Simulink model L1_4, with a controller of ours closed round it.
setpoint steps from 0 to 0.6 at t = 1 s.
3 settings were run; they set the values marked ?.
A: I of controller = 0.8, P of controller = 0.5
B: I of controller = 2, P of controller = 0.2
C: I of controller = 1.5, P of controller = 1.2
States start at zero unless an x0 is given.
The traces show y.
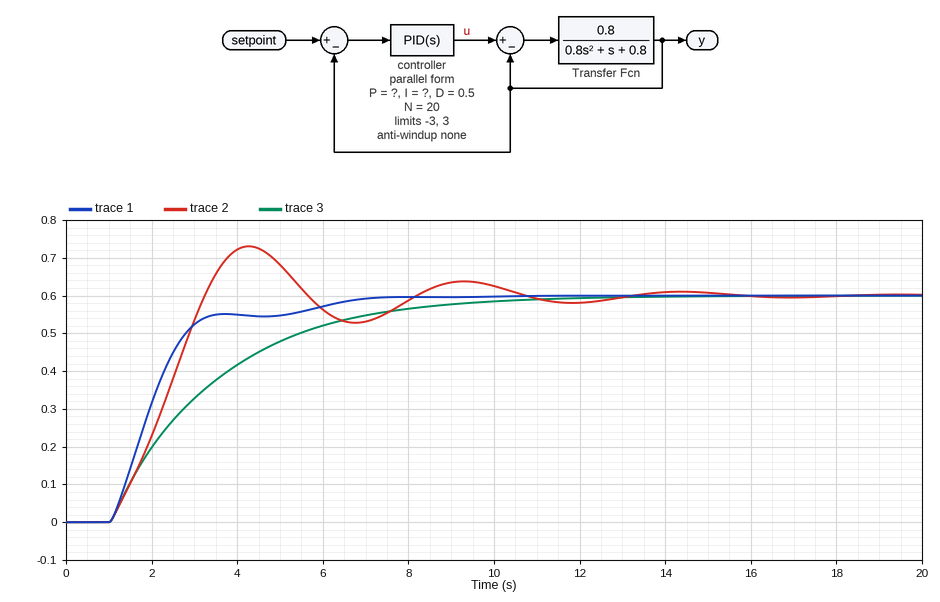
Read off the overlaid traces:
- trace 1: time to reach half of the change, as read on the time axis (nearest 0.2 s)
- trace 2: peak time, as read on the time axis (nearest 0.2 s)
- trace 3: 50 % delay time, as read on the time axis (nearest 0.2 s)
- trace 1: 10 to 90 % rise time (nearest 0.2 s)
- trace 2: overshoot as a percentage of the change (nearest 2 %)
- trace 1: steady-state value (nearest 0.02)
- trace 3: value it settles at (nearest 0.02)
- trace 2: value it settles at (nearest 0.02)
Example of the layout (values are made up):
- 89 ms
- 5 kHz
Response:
- 2.0 s
- 4.2 s
- 2.8 s
- 2.0 s
- 22 %
- 0.60
- 0.60
- 0.60
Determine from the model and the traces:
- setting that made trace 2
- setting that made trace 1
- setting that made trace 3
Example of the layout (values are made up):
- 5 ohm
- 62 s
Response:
- B
- C
- A
